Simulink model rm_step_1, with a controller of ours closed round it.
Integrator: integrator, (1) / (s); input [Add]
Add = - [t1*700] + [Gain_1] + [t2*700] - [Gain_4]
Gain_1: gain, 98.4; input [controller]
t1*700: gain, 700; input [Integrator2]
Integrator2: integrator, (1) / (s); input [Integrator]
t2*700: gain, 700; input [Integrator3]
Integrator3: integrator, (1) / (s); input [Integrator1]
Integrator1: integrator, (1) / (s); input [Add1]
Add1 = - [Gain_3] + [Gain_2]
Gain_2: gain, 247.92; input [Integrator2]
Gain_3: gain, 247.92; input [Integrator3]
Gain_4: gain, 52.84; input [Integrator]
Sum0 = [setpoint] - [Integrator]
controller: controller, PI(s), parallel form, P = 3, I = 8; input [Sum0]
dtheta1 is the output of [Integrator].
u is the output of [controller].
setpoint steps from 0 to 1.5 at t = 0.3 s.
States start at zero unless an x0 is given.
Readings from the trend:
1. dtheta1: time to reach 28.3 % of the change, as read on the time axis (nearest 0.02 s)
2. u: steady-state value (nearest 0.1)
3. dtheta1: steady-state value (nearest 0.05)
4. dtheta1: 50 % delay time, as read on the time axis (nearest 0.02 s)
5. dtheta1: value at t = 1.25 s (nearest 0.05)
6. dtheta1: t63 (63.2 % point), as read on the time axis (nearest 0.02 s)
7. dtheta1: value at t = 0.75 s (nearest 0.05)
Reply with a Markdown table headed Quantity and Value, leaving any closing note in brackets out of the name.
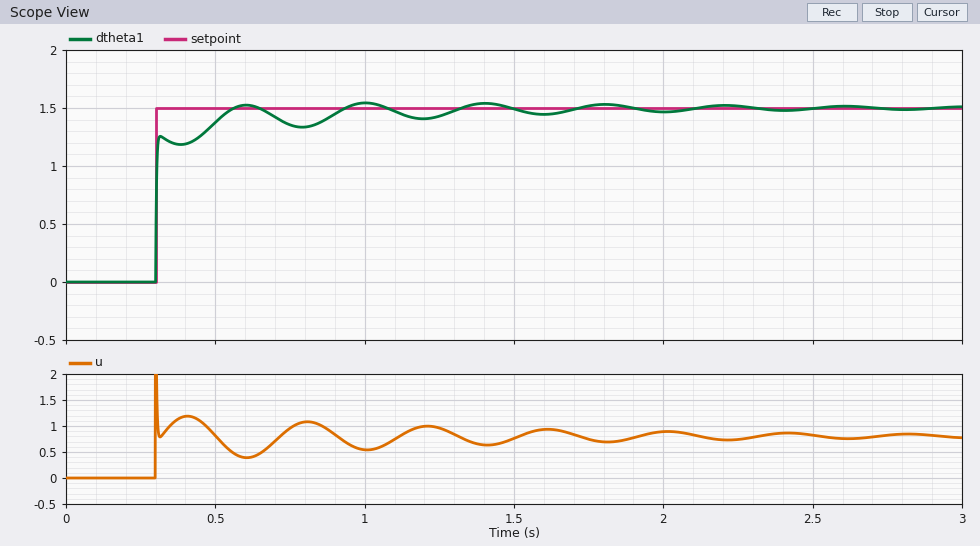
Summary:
| Quantity | Value |
|---|---|
| dtheta1: time to reach 28.3 % of the change, as read on the time axis | 0.30 s |
| u: steady-state value | 0.8 |
| dtheta1: steady-state value | 1.50 |
| dtheta1: 50 % delay time, as read on the time axis | 0.30 s |
| dtheta1: value at t = 1.25 s | 1.45 |
| dtheta1: t63 (63.2 % point), as read on the time axis | 0.30 s |
| dtheta1: value at t = 0.75 s | 1.35 |
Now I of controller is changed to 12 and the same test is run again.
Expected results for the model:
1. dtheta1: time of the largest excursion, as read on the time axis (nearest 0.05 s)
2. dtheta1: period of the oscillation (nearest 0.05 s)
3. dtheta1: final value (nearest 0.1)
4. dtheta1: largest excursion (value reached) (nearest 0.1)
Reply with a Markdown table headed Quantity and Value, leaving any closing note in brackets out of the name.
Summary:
| Quantity | Value |
|---|---|
| dtheta1: time of the largest excursion, as read on the time axis | 1.00 s |
| dtheta1: period of the oscillation | 0.40 s |
| dtheta1: final value | 1.5 |
| dtheta1: largest excursion (value reached) | 1.6 |
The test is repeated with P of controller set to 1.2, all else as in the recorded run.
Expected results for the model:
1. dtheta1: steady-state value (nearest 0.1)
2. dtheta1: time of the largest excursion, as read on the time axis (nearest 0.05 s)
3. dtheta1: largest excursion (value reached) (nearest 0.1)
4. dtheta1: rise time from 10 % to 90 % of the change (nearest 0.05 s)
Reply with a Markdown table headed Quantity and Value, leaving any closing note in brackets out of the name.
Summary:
| Quantity | Value |
|---|---|
| dtheta1: steady-state value | 1.5 |
| dtheta1: time of the largest excursion, as read on the time axis | 0.60 s |
| dtheta1: largest excursion (value reached) | 1.6 |
| dtheta1: rise time from 10 % to 90 % of the change | 0.20 s |
